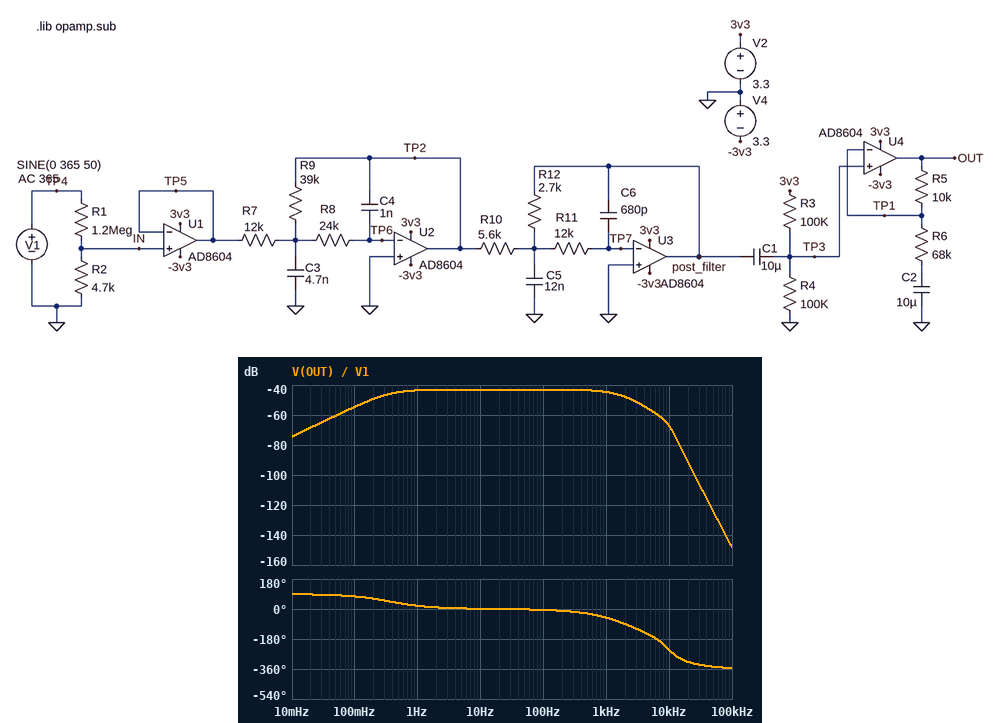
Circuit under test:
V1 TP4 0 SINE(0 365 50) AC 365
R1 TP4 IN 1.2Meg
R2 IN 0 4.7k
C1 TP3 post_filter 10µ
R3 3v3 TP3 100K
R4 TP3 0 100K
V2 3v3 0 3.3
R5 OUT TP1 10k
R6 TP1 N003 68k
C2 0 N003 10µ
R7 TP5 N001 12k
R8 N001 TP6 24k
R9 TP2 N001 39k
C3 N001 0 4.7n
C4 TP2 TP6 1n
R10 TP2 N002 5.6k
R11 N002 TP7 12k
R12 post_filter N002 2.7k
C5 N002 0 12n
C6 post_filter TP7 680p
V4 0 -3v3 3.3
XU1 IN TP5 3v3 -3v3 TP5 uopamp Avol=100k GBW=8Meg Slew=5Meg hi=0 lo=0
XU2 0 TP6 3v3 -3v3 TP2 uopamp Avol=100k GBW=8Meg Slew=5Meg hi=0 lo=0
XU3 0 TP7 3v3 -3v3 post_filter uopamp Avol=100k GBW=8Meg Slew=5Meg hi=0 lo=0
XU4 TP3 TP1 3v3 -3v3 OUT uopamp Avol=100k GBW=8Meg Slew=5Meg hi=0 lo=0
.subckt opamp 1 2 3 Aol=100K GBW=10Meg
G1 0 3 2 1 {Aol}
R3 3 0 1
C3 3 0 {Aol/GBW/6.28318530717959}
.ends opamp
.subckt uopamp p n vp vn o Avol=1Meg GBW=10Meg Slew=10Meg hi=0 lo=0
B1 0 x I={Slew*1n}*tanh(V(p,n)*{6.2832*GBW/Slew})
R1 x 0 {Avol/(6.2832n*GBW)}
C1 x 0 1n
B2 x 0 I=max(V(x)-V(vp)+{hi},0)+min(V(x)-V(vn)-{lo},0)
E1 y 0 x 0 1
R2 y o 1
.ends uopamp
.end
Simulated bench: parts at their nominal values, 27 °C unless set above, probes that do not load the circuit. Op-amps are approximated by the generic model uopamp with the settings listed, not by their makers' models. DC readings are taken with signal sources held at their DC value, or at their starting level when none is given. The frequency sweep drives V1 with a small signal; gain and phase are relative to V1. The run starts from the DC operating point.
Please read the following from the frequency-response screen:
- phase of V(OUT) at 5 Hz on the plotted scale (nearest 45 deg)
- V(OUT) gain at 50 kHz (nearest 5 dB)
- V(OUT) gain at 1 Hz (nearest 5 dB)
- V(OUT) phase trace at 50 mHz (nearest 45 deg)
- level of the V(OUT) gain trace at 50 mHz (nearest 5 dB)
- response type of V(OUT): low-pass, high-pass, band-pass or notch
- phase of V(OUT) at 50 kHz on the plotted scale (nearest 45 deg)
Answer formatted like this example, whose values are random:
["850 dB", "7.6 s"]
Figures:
["0 deg", "-125 dB", "-45 dB", "90 deg", "-60 dB", "band-pass", "-360 deg"]
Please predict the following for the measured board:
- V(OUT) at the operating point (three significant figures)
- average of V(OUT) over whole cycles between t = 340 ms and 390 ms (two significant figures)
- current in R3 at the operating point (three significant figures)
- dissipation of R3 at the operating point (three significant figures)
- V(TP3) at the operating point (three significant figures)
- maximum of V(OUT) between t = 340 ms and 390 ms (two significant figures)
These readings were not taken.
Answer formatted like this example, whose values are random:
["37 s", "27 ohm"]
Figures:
["1.65 V", "1.6 V", "16.5 µA", "27.2 µW", "1.65 V", "3.3 V"]
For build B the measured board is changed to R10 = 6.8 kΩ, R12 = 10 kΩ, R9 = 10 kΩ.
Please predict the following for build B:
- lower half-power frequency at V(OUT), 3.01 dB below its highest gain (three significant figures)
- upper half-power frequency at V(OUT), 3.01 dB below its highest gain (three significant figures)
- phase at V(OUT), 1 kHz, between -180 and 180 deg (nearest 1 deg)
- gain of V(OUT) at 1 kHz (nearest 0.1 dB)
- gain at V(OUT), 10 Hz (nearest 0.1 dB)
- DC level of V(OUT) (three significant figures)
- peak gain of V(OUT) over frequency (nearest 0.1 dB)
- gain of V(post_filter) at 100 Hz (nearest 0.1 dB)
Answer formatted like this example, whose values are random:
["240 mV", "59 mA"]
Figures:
["370 mHz", "4.86 kHz", "-30 deg", "-45.1 dB", "-45.2 dB", "1.65 V", "-44.9 dB", "-46.4 dB"]
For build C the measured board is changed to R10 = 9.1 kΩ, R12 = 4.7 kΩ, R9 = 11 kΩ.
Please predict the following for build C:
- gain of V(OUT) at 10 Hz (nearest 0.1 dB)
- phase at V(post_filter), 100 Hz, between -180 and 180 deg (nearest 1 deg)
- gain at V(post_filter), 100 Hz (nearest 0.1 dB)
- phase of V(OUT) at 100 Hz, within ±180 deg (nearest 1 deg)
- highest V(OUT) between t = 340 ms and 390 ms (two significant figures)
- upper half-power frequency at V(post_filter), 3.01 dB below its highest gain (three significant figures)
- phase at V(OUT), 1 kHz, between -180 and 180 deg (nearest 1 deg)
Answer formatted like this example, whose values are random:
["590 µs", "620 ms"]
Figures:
["-53.5 dB", "-3 deg", "-54.7 dB", "-2 deg", "2.4 V", "5.46 kHz", "-26 deg"]
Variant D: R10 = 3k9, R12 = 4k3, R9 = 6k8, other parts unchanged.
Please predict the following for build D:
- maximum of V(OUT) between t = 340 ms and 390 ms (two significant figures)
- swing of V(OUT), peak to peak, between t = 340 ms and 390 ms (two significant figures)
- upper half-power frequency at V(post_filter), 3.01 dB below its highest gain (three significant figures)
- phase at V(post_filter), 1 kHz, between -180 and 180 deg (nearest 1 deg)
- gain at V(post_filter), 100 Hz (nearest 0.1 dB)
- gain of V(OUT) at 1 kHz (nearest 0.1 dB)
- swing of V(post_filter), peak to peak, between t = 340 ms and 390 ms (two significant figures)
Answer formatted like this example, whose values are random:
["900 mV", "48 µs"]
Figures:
["2.7 V", "2.0 V", "5.92 kHz", "-23 deg", "-52.3 dB", "-51.1 dB", "1.8 V"]
